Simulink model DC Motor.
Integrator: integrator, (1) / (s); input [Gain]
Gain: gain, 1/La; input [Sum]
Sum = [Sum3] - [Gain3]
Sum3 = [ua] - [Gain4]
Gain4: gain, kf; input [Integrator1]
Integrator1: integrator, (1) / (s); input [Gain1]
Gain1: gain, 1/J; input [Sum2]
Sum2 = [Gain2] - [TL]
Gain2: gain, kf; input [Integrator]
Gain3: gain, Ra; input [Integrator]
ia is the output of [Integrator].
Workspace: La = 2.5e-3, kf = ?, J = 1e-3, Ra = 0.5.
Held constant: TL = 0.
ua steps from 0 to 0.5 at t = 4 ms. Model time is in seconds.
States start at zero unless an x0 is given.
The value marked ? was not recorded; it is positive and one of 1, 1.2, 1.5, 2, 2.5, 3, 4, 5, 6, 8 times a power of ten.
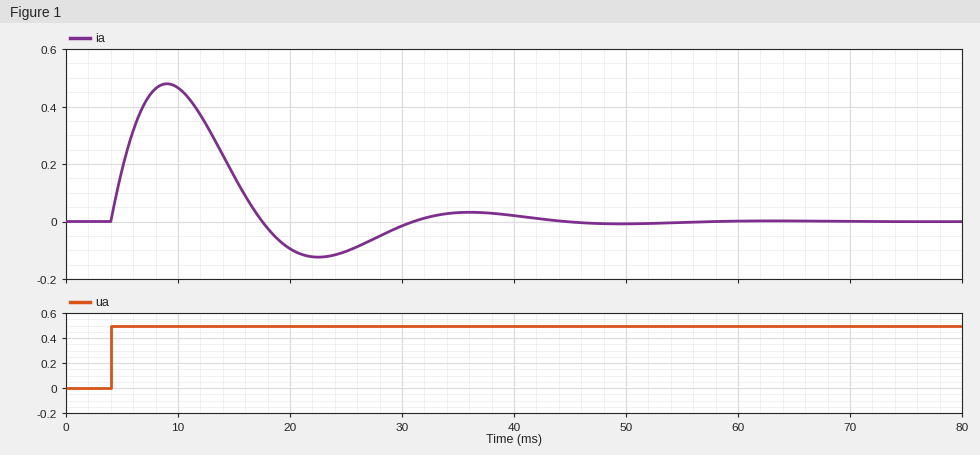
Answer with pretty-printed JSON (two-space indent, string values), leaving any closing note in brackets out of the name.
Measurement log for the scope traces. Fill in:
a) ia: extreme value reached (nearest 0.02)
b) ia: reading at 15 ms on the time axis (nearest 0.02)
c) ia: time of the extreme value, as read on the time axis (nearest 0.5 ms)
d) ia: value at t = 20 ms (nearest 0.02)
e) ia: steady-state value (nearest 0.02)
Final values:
{
  "ia: extreme value reached": "0.48",
  "ia: reading at 15 ms on the time axis": "0.16",
  "ia: time of the extreme value, as read on the time axis": "9.0 ms",
  "ia: value at t = 20 ms": "-0.10",
  "ia: steady-state value": "0.00"
}
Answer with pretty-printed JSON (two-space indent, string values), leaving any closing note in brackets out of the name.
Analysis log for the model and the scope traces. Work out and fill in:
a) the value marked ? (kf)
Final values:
{
  "the value marked ?": "0.4"
}
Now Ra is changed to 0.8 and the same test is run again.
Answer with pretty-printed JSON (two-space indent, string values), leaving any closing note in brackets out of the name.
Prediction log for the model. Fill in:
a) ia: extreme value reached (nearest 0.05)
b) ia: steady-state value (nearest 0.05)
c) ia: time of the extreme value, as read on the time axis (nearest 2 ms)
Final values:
{
  "ia: extreme value reached": "0.40",
  "ia: steady-state value": "0.00",
  "ia: time of the extreme value, as read on the time axis": "8 ms"
}
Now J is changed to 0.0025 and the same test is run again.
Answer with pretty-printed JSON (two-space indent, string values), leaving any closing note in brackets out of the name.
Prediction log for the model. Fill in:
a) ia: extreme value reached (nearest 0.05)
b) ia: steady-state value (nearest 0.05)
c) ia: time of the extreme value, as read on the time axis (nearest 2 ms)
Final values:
{
  "ia: extreme value reached": "0.60",
  "ia: steady-state value": "0.00",
  "ia: time of the extreme value, as read on the time axis": "12 ms"
}
